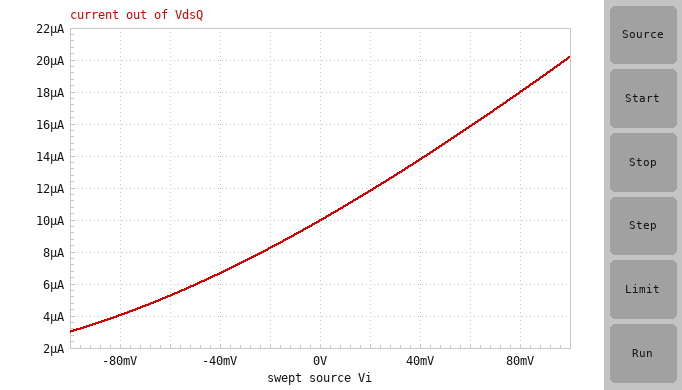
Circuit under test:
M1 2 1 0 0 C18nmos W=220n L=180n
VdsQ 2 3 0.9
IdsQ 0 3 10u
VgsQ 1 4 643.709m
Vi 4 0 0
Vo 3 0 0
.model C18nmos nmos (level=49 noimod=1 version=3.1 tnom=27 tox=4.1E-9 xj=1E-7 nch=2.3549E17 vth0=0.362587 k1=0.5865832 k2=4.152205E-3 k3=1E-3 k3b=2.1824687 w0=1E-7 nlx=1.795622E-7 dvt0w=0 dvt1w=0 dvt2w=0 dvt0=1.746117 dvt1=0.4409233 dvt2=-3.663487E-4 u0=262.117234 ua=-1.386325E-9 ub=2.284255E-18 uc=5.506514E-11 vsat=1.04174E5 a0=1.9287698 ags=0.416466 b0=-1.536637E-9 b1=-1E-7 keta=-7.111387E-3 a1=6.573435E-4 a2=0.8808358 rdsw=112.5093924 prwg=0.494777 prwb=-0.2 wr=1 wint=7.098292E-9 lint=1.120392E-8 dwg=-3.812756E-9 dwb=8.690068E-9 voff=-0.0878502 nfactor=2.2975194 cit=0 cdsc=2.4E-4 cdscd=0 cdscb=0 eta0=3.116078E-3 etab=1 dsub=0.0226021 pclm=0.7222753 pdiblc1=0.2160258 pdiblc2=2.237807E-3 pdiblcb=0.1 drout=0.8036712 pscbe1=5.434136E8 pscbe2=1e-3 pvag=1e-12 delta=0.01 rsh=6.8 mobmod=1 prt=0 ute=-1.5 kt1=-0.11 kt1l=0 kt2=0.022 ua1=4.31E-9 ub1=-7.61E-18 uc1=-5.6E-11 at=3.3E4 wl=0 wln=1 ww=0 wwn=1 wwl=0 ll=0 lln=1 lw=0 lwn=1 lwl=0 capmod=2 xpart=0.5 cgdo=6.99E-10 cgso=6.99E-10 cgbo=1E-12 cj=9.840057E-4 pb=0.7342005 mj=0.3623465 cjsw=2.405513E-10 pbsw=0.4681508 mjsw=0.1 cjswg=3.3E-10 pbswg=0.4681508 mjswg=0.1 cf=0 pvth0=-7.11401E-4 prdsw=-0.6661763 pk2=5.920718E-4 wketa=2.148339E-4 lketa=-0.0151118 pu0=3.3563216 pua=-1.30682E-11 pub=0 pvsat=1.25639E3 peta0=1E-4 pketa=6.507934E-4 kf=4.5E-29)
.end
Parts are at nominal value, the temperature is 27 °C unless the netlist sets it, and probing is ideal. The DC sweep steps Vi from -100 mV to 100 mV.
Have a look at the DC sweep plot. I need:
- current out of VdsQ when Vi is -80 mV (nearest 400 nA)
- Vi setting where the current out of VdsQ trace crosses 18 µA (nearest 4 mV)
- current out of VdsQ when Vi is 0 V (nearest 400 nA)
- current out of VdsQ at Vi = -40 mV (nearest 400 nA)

4.0 µA
80 mV
10.0 µA
6.8 µA
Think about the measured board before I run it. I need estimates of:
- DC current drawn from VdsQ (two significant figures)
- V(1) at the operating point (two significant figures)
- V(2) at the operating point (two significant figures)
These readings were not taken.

10 µA
640 mV
900 mV
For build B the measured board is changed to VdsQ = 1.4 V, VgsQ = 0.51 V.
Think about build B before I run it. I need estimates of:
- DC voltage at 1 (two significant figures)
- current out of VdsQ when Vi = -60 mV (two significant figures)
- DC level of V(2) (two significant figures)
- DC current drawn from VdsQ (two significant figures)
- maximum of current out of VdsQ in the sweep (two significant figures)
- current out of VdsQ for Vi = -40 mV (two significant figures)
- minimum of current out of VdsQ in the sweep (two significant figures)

510 mV
740 nA
1.4 V
2.3 µA
8.6 µA
1.1 µA
310 nA
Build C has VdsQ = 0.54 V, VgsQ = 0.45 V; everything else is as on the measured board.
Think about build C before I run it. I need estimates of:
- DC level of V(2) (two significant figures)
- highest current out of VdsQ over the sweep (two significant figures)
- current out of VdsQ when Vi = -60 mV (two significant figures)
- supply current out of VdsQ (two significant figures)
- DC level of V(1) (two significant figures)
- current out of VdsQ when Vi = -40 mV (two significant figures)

540 mV
2.8 µA
100 nA
400 nA
450 mV
160 nA
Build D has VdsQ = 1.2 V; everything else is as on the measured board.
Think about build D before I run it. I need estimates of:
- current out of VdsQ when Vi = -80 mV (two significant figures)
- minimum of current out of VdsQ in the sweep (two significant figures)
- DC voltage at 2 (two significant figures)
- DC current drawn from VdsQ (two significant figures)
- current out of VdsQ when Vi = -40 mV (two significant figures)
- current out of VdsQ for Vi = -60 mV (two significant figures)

4.6 µA
3.5 µA
1.2 V
11 µA
7.5 µA
6.0 µA
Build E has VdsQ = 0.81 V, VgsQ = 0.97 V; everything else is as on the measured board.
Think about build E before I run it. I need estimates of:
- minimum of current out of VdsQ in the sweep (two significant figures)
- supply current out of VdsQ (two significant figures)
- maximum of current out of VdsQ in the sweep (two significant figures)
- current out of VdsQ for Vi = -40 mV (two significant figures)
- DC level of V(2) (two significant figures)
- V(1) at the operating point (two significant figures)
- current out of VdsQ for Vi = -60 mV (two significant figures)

35 µA
48 µA
62 µA
43 µA
810 mV
970 mV
40 µA
